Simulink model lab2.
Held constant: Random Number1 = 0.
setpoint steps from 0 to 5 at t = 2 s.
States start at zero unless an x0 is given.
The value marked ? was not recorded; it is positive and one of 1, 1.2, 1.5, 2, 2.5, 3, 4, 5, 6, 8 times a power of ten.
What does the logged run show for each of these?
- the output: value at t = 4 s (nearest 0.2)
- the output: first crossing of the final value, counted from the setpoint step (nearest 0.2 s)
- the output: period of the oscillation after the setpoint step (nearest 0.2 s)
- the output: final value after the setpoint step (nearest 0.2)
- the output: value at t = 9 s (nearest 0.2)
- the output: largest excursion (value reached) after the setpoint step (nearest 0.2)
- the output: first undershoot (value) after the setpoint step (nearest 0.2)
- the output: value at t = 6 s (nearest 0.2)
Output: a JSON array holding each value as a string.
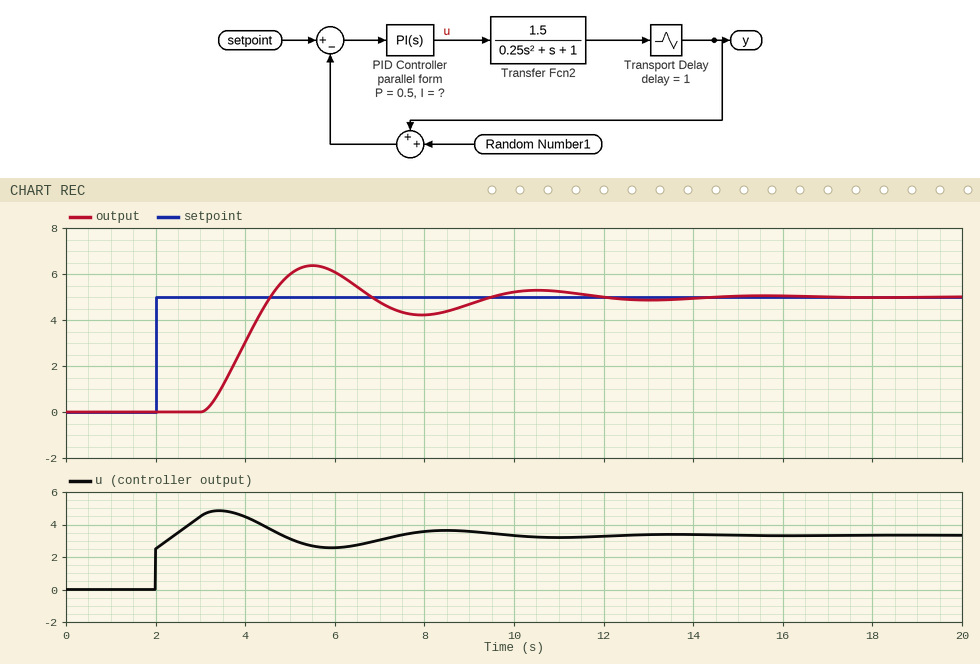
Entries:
["3.0", "2.6 s", "5.0 s", "5.0", "4.6", "6.4", "4.2", "6.0"]
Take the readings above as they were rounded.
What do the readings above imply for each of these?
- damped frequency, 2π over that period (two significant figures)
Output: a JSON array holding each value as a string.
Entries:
["1.3 rad/s"]
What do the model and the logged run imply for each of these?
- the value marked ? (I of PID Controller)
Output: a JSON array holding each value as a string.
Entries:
["0.4"]
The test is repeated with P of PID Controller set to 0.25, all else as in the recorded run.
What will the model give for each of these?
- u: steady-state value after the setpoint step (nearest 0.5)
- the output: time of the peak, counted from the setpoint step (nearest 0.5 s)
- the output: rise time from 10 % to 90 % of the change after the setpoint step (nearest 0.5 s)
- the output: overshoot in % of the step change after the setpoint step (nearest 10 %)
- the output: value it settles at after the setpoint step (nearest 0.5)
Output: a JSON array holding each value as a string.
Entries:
["3.5", "4.5 s", "1.5 s", "30 %", "5.0"]
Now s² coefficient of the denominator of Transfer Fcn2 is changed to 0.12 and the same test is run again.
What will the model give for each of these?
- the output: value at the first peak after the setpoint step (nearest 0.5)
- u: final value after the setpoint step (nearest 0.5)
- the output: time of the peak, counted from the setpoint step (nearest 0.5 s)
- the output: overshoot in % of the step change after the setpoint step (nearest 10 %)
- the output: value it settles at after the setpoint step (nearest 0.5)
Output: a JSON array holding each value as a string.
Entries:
["6.0", "3.5", "3.5 s", "20 %", "5.0"]
